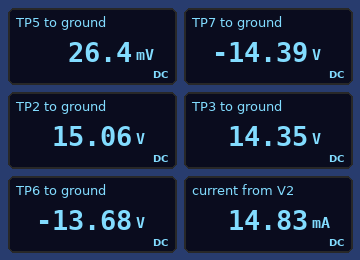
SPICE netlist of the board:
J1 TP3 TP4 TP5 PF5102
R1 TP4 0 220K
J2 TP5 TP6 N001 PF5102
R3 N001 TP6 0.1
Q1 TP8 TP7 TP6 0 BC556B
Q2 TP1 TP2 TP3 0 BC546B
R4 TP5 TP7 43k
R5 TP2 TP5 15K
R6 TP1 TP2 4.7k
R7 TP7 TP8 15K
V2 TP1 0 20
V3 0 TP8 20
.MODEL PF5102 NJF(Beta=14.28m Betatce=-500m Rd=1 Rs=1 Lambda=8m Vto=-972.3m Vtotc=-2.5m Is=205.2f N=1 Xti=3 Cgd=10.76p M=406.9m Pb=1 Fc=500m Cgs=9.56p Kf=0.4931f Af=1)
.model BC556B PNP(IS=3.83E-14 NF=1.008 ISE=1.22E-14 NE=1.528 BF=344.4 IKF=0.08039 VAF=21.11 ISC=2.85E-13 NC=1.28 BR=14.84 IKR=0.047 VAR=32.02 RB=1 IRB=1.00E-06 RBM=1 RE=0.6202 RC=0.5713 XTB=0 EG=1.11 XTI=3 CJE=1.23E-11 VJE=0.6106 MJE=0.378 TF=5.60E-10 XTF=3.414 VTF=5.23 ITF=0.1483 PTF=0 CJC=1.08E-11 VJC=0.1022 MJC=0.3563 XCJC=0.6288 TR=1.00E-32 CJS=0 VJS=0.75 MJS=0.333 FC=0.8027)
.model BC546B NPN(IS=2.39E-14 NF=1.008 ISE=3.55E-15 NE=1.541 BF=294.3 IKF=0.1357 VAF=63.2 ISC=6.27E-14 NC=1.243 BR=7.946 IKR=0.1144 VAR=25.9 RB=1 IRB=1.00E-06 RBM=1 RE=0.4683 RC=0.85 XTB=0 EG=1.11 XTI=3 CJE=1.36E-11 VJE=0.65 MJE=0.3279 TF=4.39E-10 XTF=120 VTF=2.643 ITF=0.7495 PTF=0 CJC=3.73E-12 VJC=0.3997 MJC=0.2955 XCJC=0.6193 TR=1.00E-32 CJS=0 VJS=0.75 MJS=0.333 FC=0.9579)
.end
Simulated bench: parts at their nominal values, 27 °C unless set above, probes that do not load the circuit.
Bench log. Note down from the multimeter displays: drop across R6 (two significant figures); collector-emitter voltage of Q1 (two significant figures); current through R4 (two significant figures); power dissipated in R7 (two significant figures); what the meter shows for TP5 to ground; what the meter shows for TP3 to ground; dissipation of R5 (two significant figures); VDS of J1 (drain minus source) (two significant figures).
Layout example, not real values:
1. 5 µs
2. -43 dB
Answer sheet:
1. 4.9 V
2. -6.3 V
3. 340 µA
4. 2.1 mW
5. 26.4 mV
6. 14.35 V
7. 15 mW
8. 14 V
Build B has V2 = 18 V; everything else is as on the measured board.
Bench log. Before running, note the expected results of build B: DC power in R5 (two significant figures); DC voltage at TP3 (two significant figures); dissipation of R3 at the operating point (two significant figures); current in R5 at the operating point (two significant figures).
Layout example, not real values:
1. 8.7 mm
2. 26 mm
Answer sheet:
1. 12 mW
2. 13 V
3. 21 µW
4. 900 µA
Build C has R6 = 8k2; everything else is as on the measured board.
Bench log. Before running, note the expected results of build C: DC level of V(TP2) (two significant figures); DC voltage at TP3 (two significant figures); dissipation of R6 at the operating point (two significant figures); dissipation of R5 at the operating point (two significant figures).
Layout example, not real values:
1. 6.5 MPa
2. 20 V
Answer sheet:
1. 13 V
2. 12 V
3. 6.5 mW
4. 11 mW
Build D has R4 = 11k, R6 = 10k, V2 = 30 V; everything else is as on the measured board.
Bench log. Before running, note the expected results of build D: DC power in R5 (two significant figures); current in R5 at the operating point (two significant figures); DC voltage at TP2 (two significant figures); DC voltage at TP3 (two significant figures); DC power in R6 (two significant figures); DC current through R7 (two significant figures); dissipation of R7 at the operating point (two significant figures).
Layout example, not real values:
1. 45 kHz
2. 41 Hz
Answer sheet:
1. 21 mW
2. 1.2 mA
3. 18 V
4. 17 V
5. 15 mW
6. 780 µA
7. 9.2 mW
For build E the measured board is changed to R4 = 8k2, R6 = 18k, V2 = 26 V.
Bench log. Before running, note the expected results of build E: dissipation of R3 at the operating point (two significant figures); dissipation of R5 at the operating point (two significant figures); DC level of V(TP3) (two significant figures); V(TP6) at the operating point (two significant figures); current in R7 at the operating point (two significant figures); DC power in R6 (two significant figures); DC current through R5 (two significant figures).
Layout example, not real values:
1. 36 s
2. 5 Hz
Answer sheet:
1. 19 µW
2. 8.8 mW
3. 11 V
4. -6.2 V
5. 870 µA
6. 12 mW
7. 760 µA
